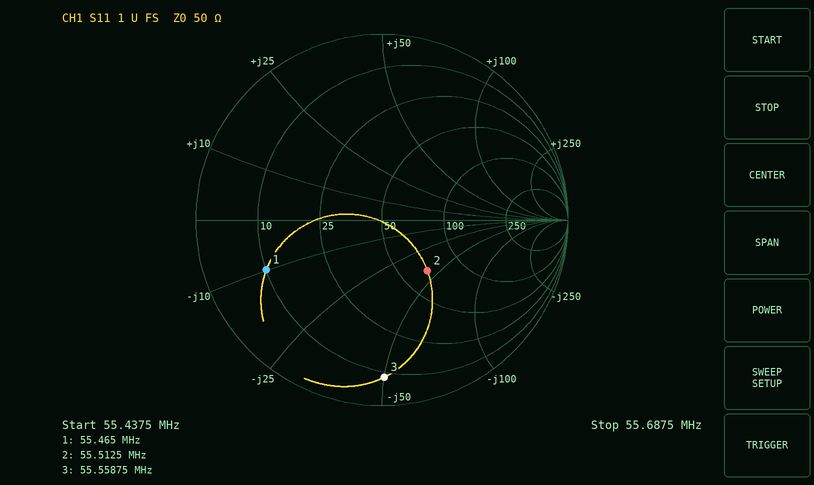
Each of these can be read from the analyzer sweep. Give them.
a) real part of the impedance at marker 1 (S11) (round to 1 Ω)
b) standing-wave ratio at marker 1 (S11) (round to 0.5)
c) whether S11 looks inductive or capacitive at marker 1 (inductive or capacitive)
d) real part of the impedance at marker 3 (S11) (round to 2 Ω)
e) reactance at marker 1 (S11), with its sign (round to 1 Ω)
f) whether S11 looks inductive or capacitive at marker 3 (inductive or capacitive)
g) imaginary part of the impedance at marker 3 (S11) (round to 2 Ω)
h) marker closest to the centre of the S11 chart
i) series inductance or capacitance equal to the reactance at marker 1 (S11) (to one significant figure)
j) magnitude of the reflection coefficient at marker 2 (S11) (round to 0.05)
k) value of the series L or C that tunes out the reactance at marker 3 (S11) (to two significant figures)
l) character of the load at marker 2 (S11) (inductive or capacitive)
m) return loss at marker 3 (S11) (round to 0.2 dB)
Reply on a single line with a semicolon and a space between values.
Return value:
10 Ω; 5.0; capacitive; 8 Ω; -10 Ω; capacitive; -50 Ω; marker 2; 300 pF; 0.35; 140 nH; capacitive; 1.4 dB
